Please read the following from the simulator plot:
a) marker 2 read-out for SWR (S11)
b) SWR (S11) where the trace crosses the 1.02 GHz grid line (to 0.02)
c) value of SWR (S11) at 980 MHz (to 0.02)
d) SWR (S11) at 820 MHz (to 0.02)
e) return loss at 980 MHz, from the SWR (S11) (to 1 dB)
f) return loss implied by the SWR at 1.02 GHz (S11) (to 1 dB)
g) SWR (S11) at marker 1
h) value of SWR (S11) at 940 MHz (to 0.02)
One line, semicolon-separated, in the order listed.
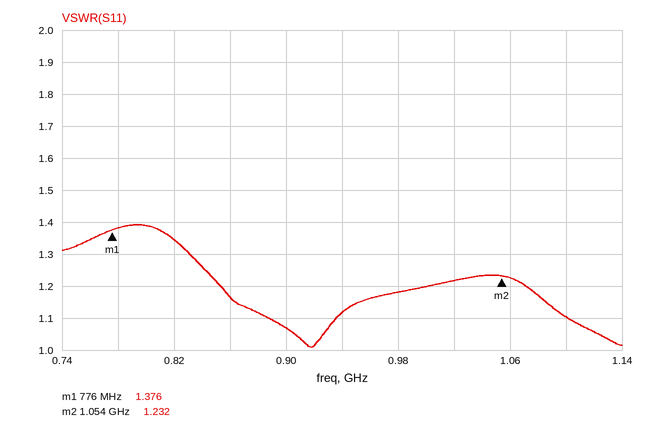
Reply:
1.232; 1.22; 1.18; 1.34; 22 dB; 20 dB; 1.376; 1.12
